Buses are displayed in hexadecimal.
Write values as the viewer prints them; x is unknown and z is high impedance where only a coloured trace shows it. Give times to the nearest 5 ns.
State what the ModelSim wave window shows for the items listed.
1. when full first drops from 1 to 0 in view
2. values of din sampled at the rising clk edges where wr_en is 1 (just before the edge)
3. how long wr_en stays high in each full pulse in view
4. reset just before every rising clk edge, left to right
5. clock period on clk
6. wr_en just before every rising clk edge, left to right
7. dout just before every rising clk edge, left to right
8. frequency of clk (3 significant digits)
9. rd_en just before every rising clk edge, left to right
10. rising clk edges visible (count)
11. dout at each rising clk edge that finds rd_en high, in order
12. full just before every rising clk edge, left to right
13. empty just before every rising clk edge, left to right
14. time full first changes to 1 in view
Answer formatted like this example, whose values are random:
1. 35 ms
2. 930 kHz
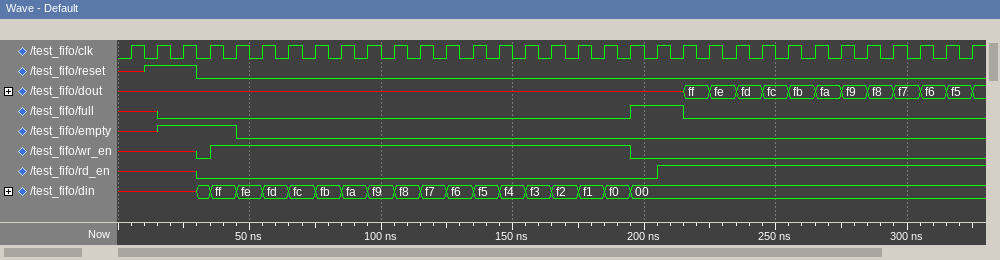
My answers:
1. 215 ns
2. ff, fe, fd, fc, fb, fa, f9, f8, f7, f6, f5, f4, f3, f2, f1, f0
3. 160 ns
4. x 1 1 0 0 0 0 0 0 0 0 0 0 0 0 0 0 0 0 0 0 0 0 0 0 0 0 0 0 0 0 0 0
5. 10 ns
6. x x x 0 1 1 1 1 1 1 1 1 1 1 1 1 1 1 1 1 0 0 0 0 0 0 0 0 0 0 0 0 0
7. x, x, x, x, x, x, x, x, x, x, x, x, x, x, x, x, x, x, x, x, x, x, ff, fe, fd, fc, fb, fa, f9, f8, f7, f6, f5
8. 100 MHz
9. x x x 0 0 0 0 0 0 0 0 0 0 0 0 0 0 0 0 0 0 1 1 1 1 1 1 1 1 1 1 1 1
10. 33
11. x, ff, fe, fd, fc, fb, fa, f9, f8, f7, f6, f5
12. x x 0 0 0 0 0 0 0 0 0 0 0 0 0 0 0 0 0 0 1 1 0 0 0 0 0 0 0 0 0 0 0
13. x x 1 1 1 0 0 0 0 0 0 0 0 0 0 0 0 0 0 0 0 0 0 0 0 0 0 0 0 0 0 0 0
14. 195 ns
